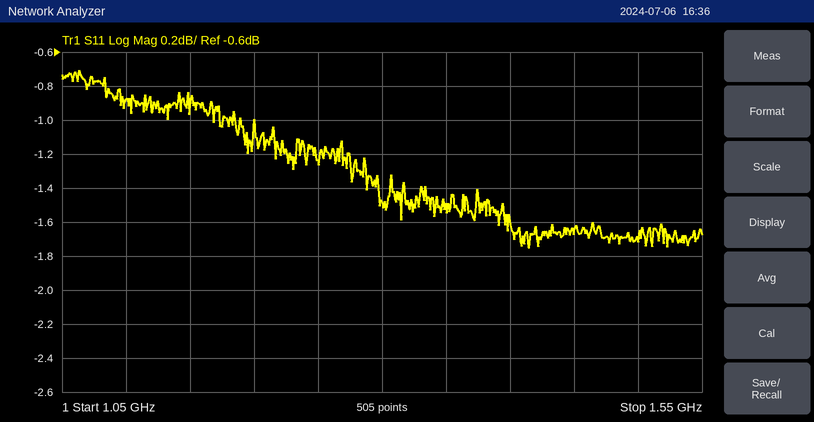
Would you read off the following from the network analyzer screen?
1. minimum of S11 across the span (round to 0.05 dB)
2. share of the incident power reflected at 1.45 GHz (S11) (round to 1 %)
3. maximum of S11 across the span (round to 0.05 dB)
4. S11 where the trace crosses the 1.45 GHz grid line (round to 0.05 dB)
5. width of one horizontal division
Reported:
-1.75 dB
68 %
-0.70 dB
-1.65 dB
50 MHz
